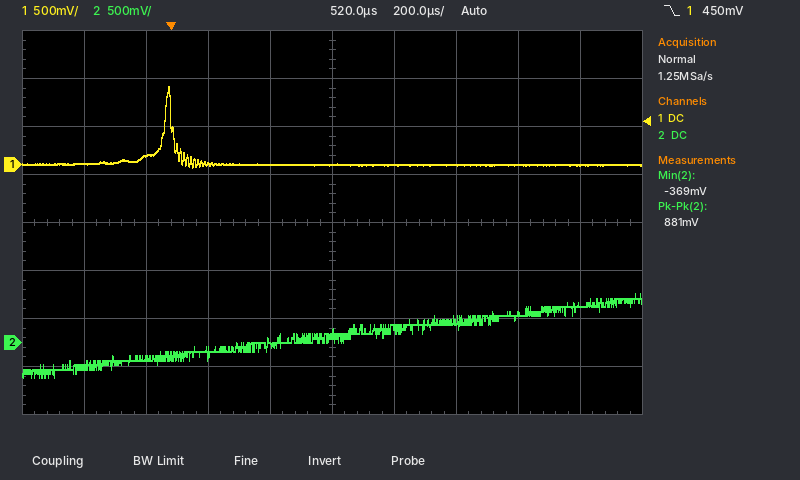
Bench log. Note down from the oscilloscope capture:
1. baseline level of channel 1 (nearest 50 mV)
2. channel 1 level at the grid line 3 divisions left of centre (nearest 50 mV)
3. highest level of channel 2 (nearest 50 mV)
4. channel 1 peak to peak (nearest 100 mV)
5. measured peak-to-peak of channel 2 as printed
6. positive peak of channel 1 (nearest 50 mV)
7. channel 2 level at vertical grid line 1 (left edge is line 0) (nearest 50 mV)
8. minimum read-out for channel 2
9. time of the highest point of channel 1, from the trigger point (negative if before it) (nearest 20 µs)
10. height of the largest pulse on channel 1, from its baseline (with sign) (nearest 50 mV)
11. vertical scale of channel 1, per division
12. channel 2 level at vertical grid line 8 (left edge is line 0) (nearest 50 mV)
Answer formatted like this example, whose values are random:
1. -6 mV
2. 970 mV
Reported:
1. 0 mV
2. 100 mV
3. 500 mV
4. 800 mV
5. 881 mV
6. 800 mV
7. -250 mV
8. -369 mV
9. 0 µs
10. +800 mV
11. 500 mV
12. 300 mV
